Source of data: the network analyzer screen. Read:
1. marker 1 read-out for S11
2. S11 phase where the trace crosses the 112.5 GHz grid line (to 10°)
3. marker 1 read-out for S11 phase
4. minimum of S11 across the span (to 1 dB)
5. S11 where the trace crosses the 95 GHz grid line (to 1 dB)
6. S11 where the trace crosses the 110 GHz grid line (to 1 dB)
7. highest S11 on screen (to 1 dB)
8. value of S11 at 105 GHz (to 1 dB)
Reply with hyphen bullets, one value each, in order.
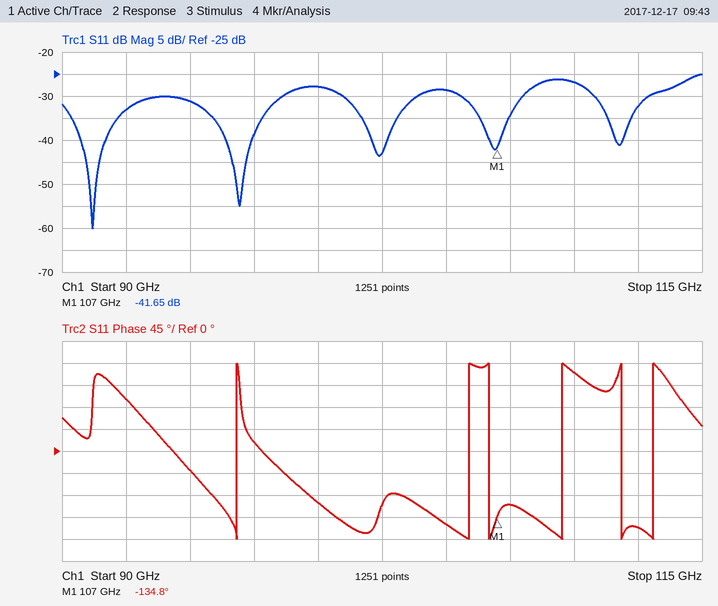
- -41.65 dB
- -160°
- -134.8°
- -60 dB
- -31 dB
- -27 dB
- -25 dB
- -29 dB
